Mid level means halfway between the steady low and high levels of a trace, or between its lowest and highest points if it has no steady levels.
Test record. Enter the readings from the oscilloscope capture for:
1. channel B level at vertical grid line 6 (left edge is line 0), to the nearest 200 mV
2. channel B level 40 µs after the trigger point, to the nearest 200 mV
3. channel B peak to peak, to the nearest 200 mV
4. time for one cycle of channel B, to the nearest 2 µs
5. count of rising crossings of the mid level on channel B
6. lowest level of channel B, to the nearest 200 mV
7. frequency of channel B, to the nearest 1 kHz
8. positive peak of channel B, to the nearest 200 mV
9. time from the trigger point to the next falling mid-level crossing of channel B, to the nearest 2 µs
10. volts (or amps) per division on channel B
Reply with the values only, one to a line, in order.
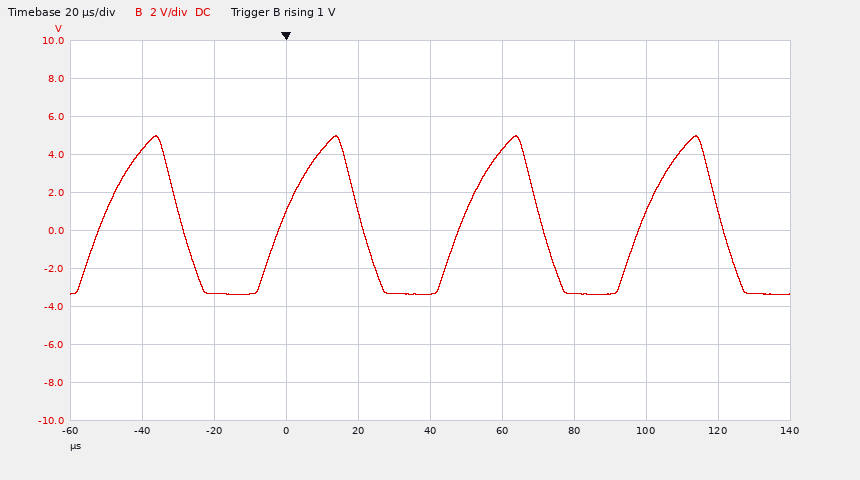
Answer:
4.2 V
-3.4 V
8.4 V
50 µs
4
-3.4 V
20 kHz
5.0 V
20 µs
2 V
